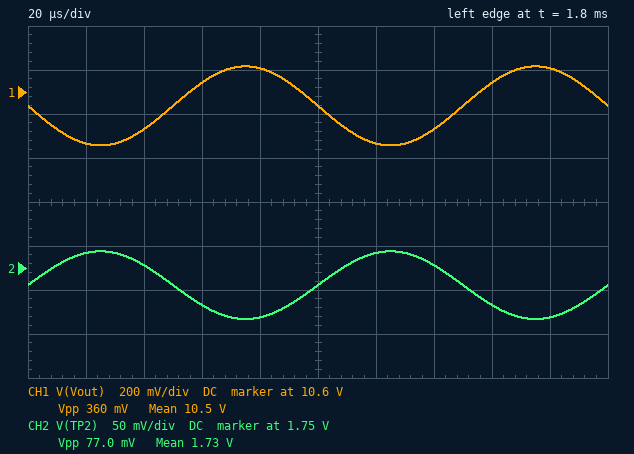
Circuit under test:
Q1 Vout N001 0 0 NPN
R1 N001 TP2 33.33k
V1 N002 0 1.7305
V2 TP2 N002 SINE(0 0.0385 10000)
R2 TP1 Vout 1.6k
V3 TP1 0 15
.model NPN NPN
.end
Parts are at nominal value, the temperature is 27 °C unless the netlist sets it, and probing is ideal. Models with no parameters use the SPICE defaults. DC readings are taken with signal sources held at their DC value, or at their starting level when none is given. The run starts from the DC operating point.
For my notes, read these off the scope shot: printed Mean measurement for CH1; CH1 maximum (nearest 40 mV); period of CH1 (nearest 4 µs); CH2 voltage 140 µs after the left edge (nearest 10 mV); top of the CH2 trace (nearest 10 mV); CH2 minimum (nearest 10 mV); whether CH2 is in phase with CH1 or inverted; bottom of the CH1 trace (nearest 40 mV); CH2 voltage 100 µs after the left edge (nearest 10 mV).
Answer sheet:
10.5 V
10.72 V
100 µs
1.75 V
1.77 V
1.69 V
inverted
10.36 V
1.73 V
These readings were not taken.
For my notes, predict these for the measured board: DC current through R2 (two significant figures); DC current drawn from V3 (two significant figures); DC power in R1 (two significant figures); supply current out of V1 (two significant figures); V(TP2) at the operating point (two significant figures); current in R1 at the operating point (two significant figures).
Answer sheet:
2.8 mA
2.8 mA
26 µW
28 µA
1.7 V
28 µA
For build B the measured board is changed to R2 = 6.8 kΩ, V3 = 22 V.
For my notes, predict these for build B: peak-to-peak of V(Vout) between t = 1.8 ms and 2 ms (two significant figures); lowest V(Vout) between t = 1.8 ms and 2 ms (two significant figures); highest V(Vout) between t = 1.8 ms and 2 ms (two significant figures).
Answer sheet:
1.5 V
2.3 V
3.8 V
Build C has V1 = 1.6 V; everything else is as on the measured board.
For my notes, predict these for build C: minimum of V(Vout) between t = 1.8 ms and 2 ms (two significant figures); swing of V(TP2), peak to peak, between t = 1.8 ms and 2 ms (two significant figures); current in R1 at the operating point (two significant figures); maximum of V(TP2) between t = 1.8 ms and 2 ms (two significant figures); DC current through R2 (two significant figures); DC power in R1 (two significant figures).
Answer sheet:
11 V
77 mV
24 µA
1.6 V
2.4 mA
19 µW
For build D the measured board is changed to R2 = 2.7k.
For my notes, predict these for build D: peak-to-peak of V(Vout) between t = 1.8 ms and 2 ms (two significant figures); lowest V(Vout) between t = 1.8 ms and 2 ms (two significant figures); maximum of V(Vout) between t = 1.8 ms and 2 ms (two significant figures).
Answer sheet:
610 mV
7.2 V
7.8 V
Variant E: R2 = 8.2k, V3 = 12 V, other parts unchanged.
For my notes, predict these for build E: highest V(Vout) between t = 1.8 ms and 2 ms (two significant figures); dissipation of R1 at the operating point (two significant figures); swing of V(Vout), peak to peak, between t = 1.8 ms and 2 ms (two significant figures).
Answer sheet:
120 mV
27 µW
4.2 mV
